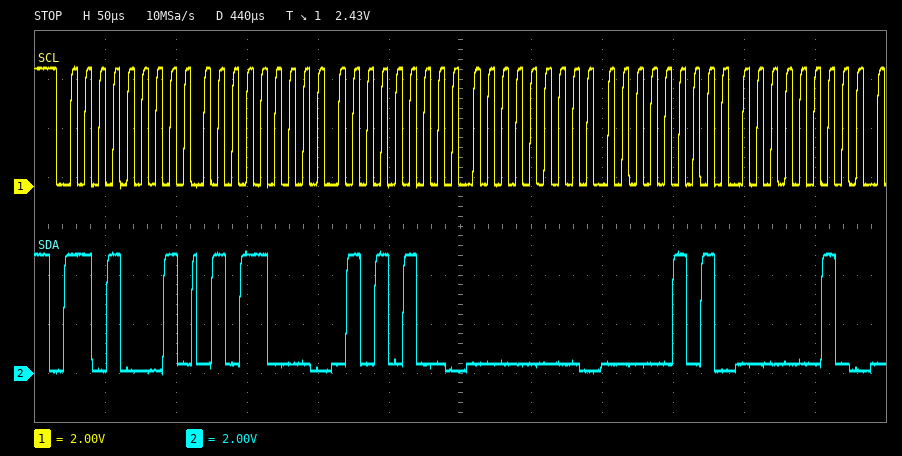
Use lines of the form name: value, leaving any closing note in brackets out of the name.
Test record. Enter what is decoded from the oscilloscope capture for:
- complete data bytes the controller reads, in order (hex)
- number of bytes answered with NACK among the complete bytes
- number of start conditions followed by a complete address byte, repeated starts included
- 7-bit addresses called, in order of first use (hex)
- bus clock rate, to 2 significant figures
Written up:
complete data bytes the controller reads, in order: 58 54 00 05 02
number of bytes answered with NACK among the complete bytes: 0
number of start conditions followed by a complete address byte, repeated starts included: 1
7-bit addresses called, in order of first use: 0x68
bus clock rate, to 2 significant figures: 100 kHz
